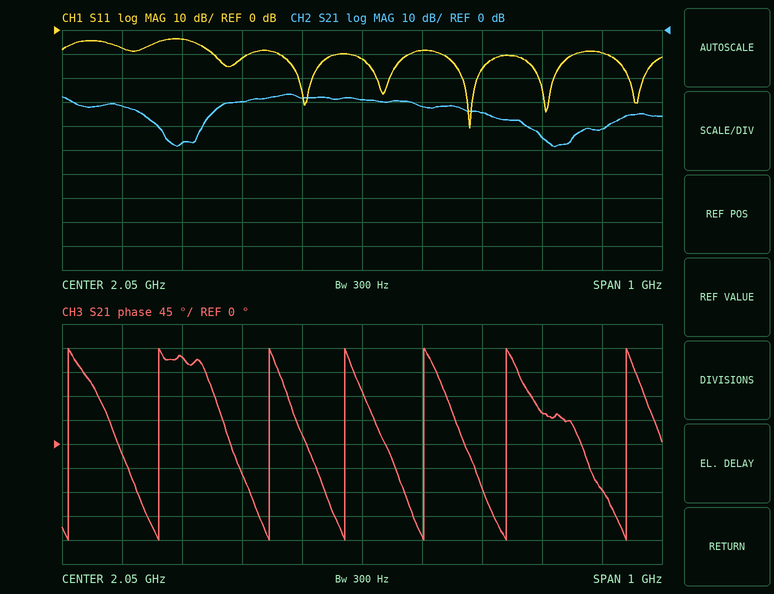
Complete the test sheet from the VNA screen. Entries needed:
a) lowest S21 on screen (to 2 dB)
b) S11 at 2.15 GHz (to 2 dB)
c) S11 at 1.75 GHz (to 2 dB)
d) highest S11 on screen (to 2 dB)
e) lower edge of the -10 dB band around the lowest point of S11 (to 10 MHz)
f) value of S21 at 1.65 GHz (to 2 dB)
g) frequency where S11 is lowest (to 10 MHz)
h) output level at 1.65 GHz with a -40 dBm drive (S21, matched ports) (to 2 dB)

-48 dB
-8 dB
-4 dB
-4 dB
2.18 GHz
-32 dB
2.23 GHz
-72 dBm
